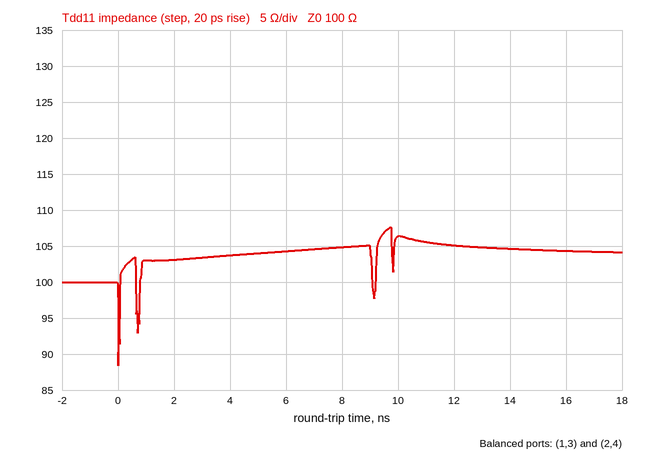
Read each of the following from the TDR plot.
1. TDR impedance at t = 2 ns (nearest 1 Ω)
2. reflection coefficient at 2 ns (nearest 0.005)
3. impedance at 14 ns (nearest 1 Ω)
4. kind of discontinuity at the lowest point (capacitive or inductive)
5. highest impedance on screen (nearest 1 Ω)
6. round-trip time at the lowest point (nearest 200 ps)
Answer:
103 Ω
+0.015
105 Ω
capacitive
108 Ω
0.0 ns
